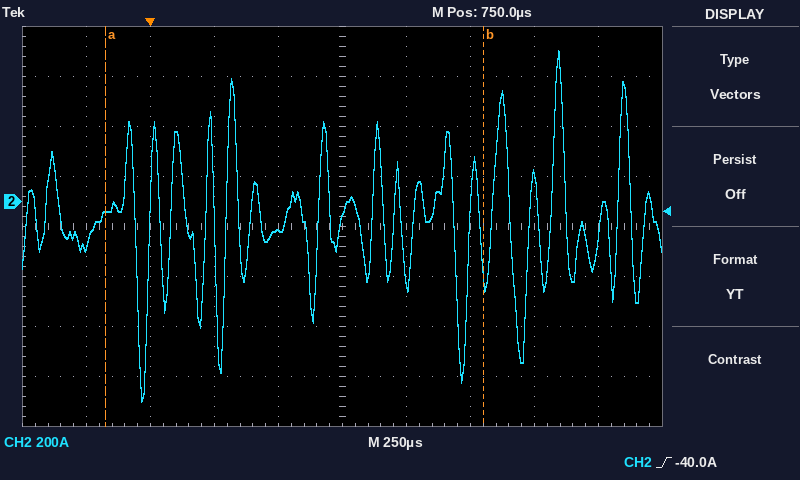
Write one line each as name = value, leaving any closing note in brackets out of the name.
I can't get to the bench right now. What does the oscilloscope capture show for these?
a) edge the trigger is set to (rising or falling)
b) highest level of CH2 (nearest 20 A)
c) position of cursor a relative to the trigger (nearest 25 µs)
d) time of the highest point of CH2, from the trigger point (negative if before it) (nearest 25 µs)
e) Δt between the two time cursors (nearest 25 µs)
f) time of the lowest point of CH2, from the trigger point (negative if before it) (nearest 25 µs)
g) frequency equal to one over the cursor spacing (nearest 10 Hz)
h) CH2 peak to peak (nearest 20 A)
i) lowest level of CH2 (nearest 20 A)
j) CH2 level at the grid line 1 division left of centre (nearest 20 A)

edge the trigger is set to = rising
highest level of CH2 = 600 A
position of cursor a relative to the trigger = -175 µs
time of the highest point of CH2, from the trigger point (negative if before it) = +1.600 ms
Δt between the two time cursors = 1.475 ms
time of the lowest point of CH2, from the trigger point (negative if before it) = -25 µs
frequency equal to one over the cursor spacing = 680 Hz
CH2 peak to peak = 1.40 kA
lowest level of CH2 = -800 A
CH2 level at the grid line 1 division left of centre = -120 A
